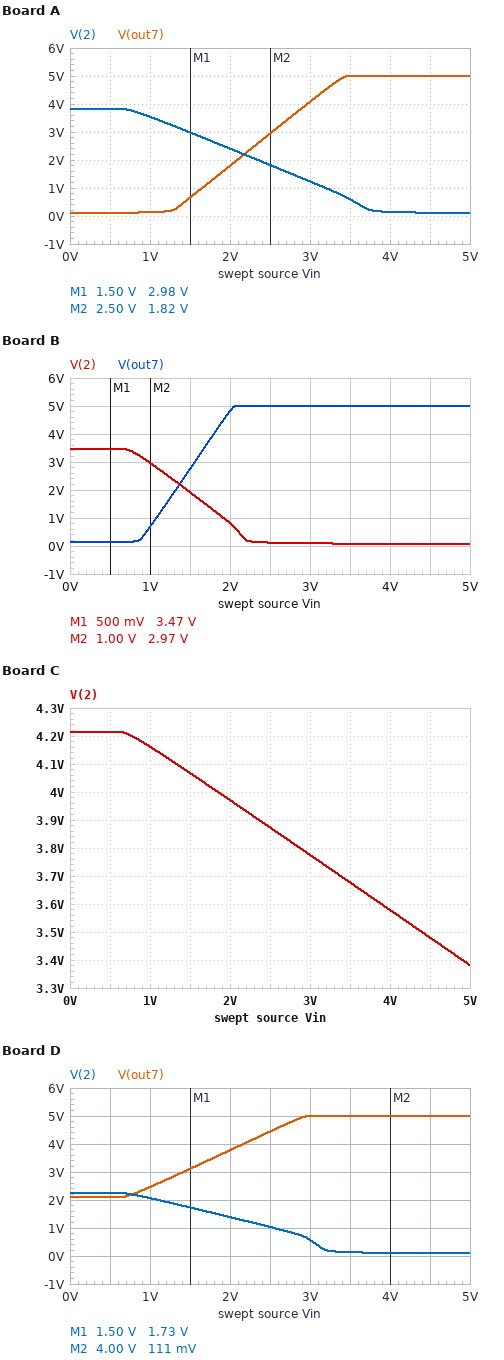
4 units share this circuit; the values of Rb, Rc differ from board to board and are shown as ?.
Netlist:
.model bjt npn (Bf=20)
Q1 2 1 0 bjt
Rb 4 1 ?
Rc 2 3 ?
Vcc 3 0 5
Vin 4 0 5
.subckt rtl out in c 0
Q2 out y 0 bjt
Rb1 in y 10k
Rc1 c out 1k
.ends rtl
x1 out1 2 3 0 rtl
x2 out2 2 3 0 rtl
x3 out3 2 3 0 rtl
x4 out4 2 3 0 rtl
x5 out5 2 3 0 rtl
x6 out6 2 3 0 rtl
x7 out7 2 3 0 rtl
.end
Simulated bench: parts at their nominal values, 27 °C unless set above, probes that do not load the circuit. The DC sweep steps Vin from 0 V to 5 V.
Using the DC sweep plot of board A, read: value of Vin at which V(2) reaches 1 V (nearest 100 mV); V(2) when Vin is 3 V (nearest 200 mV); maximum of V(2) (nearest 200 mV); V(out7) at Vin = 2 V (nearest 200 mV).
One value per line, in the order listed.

3.2 V
1.2 V
3.8 V
1.8 V
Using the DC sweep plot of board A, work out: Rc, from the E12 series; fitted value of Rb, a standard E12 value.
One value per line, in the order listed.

560 Ω
6.8 kΩ
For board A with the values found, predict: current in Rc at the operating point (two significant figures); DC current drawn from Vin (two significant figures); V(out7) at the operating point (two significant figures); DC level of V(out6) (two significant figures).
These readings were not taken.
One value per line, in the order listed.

8.7 mA
610 µA
5.0 V
5.0 V
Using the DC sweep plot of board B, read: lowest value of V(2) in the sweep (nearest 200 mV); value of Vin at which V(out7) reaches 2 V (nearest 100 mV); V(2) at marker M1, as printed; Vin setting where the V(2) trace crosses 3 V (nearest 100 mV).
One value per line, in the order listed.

0 V
1.3 V
3.47 V
1.0 V
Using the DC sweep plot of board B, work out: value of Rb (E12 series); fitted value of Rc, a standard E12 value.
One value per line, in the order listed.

4.7 kΩ
820 Ω
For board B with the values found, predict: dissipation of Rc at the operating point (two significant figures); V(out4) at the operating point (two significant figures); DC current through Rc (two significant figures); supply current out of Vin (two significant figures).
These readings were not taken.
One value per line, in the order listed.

30 mW
5.0 V
6.0 mA
890 µA
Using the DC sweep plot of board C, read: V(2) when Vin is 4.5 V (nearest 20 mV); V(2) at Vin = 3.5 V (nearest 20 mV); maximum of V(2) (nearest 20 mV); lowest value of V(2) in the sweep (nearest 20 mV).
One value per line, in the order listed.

3.48 V
3.68 V
4.22 V
3.38 V
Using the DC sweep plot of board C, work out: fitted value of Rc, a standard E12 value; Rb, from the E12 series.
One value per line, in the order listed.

330 Ω
27 kΩ
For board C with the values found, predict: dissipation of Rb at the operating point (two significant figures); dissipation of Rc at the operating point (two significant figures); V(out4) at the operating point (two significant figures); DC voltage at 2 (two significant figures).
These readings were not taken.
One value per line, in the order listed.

650 µW
7.9 mW
150 mV
3.4 V
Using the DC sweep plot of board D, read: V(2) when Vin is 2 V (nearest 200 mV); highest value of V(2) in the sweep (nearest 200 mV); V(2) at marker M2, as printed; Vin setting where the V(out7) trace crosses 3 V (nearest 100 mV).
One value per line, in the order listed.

1.4 V
2.2 V
111 mV
1.4 V
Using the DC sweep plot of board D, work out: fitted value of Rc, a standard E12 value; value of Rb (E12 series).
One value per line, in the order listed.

2.7 kΩ
27 kΩ
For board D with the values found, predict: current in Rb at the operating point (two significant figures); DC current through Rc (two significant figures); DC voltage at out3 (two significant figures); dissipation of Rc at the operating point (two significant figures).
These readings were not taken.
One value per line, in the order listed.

160 µA
1.8 mA
5.0 V
8.9 mW
